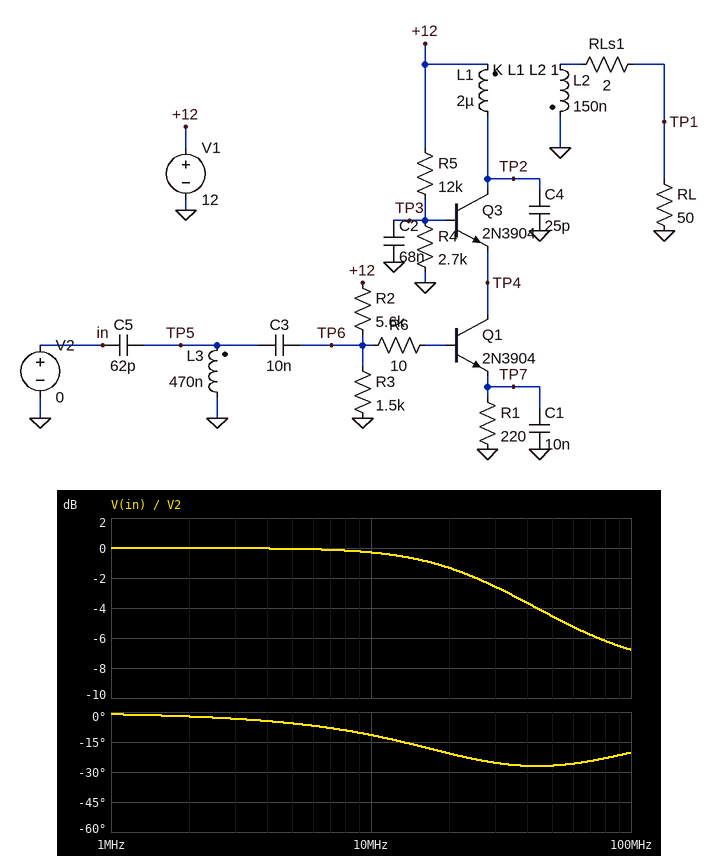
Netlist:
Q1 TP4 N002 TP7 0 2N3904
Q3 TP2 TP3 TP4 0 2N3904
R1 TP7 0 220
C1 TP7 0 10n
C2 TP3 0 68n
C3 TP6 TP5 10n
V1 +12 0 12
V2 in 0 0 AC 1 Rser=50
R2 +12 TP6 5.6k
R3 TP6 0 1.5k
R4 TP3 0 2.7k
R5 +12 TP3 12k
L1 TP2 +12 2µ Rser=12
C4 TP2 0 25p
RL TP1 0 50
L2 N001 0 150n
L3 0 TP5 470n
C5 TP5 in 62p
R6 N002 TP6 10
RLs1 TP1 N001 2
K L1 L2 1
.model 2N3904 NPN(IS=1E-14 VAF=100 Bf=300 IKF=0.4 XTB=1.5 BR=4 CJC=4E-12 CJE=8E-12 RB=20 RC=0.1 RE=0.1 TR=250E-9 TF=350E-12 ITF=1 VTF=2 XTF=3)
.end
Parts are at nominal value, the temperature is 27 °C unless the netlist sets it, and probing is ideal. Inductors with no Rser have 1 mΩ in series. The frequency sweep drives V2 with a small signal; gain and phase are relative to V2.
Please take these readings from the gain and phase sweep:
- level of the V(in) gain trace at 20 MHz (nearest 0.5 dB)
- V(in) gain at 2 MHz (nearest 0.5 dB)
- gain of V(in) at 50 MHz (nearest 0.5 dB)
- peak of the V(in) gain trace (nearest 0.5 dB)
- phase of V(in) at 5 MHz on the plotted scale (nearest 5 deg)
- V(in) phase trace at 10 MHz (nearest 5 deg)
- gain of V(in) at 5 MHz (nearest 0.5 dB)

-1.5 dB
0 dB
-4.5 dB
0 dB
-5 deg
-10 deg
0 dB
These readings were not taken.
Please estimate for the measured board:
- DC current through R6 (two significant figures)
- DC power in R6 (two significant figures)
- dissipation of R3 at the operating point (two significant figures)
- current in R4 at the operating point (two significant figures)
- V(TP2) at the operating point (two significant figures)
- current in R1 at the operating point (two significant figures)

340 µA
1.2 µW
3.0 mW
800 µA
12 V
6.4 mA
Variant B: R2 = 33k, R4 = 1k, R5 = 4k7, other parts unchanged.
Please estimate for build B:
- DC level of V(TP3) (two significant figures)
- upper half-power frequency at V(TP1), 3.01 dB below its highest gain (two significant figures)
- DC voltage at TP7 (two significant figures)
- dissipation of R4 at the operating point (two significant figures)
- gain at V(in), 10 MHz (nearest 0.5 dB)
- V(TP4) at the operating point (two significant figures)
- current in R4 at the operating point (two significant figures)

2.1 V
30 MHz
1.2 mV
4.4 mW
0 dB
1.6 V
2.1 mA
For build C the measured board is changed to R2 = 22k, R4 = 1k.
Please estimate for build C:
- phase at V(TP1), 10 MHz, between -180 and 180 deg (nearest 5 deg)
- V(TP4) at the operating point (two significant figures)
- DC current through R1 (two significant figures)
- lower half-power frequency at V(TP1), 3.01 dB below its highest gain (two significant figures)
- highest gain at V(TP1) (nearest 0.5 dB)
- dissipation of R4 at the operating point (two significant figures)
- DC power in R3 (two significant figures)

50 deg
280 mV
560 µA
19 MHz
13.0 dB
850 µW
390 µW
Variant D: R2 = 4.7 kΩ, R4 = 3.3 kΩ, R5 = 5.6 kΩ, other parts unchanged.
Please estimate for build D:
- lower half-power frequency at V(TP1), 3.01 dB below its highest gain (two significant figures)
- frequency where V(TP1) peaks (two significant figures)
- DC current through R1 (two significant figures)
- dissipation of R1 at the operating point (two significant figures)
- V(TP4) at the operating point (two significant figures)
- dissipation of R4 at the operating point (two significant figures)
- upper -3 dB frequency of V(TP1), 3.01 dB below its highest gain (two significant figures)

15 MHz
17 MHz
9.8 mA
21 mW
3.7 V
5.8 mW
22 MHz
